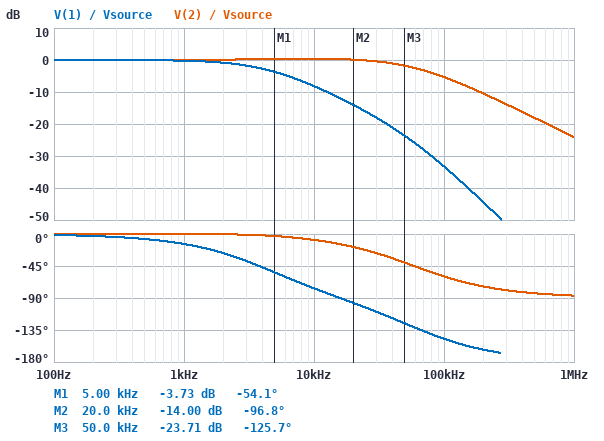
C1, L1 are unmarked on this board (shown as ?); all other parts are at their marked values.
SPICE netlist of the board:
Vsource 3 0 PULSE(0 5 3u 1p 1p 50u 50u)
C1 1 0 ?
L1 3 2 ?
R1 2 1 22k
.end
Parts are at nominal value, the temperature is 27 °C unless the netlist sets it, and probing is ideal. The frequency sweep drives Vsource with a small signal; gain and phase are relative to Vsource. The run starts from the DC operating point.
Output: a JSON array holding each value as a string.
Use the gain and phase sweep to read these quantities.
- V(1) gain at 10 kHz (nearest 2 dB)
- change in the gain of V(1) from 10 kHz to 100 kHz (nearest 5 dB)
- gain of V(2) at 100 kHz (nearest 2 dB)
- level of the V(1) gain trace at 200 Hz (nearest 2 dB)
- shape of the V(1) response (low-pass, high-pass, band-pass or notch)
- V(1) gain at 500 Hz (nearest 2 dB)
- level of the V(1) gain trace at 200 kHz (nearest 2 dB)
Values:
["-8 dB", "-25 dB", "-6 dB", "0 dB", "low-pass", "0 dB", "-44 dB"]
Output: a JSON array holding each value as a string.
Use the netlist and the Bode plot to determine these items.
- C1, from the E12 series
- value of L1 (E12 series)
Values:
["1.8 nF", "56 mH"]
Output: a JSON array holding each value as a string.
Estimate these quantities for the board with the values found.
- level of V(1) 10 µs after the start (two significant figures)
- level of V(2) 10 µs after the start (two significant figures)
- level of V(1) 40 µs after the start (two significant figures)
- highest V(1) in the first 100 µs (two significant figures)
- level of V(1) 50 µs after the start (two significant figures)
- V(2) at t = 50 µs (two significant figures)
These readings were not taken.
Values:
["560 mV", "4.9 V", "3.0 V", "4.6 V", "3.5 V", "5.1 V"]
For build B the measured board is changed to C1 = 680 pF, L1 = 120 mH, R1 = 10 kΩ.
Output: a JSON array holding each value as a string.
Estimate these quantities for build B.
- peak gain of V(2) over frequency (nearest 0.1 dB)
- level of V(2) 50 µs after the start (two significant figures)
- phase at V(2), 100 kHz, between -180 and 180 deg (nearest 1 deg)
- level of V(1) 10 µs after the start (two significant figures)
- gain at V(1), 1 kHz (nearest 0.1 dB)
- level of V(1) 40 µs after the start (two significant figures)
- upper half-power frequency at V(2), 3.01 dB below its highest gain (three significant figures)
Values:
["4.7 dB", "4.6 V", "-95 deg", "1.2 V", "0 dB", "6.1 V", "22.4 kHz"]
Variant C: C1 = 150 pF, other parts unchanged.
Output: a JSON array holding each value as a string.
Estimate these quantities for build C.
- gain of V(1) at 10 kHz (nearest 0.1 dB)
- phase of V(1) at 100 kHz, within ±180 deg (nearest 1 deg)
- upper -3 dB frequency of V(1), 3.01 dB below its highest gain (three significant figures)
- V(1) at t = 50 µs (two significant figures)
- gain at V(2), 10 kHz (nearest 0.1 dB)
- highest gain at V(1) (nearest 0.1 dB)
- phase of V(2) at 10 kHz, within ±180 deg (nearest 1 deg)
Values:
["0.1 dB", "-138 deg", "62.3 kHz", "5.0 V", "0.3 dB", "0.6 dB", "0 deg"]
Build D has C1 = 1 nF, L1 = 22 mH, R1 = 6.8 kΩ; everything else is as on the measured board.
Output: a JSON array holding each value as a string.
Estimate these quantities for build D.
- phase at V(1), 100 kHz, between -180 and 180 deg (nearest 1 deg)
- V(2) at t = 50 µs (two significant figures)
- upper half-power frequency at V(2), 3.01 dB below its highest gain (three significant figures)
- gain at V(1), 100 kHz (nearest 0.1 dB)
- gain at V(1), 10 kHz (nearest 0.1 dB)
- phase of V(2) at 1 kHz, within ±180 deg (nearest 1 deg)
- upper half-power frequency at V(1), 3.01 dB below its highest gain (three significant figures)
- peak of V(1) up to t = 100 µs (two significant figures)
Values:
["-151 deg", "5.0 V", "55.1 kHz", "-18.9 dB", "-0.1 dB", "0 deg", "33.1 kHz", "5.2 V"]
